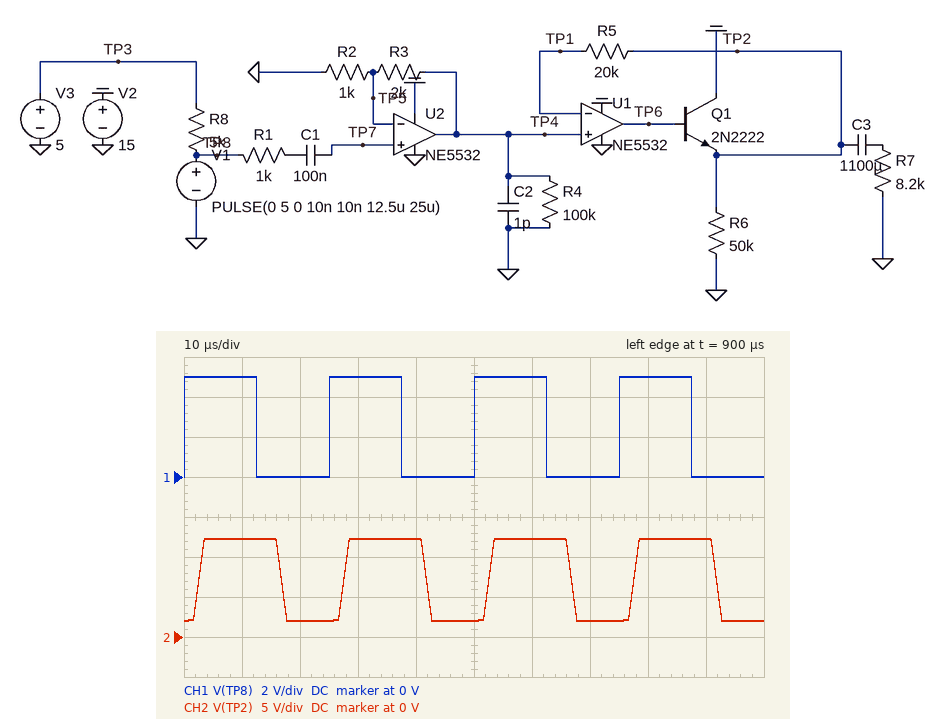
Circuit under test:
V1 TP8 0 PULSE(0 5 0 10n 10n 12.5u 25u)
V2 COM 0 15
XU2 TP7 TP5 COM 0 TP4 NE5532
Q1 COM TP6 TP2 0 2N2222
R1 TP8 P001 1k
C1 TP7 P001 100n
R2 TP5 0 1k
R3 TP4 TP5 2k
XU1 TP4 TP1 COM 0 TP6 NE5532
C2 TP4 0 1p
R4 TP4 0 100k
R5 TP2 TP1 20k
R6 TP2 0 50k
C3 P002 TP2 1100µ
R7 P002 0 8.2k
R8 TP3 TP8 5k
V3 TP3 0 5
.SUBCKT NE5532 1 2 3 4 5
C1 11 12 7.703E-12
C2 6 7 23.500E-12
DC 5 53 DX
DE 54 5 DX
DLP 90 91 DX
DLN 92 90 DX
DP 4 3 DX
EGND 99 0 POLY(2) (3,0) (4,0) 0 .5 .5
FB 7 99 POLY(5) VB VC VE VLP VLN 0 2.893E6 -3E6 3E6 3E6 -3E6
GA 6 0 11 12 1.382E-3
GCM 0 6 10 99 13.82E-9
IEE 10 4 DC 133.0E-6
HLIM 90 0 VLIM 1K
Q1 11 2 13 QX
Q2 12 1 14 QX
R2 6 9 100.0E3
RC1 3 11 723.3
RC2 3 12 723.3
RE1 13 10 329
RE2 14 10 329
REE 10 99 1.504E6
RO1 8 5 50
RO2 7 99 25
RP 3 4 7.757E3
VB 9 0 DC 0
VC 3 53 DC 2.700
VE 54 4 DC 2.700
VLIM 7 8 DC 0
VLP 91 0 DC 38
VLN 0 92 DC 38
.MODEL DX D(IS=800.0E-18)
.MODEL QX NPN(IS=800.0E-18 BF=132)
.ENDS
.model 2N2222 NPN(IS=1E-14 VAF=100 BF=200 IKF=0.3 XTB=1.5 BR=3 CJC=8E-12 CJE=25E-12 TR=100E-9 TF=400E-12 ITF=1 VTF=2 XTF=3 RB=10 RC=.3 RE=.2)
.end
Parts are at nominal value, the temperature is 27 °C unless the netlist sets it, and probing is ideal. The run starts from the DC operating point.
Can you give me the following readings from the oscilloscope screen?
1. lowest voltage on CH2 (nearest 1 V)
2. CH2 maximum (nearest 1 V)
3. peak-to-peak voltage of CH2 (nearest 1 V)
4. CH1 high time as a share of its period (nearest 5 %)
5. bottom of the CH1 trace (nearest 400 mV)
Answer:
2 V
12 V
10 V
50 %
0 V
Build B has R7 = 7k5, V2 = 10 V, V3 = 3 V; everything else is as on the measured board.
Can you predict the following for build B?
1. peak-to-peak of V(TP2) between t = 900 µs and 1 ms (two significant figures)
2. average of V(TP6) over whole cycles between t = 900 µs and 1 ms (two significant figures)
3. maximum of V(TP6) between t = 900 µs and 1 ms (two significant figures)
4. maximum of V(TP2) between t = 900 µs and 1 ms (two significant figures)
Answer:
5.3 V
5.7 V
8.0 V
7.3 V
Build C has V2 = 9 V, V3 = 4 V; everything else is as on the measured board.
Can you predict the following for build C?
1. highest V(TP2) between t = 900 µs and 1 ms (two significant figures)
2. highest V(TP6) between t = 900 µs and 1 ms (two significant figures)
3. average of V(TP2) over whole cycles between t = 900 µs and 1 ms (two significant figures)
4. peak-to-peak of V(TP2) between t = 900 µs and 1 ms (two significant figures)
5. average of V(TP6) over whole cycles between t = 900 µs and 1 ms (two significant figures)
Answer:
6.3 V
7.0 V
4.5 V
4.3 V
5.1 V
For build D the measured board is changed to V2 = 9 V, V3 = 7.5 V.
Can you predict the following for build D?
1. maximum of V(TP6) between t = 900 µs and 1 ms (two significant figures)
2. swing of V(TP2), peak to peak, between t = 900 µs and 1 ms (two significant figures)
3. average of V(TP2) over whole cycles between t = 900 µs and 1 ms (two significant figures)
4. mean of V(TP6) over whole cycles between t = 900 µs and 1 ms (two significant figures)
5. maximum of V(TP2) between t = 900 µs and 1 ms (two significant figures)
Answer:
7.0 V
4.3 V
4.5 V
5.1 V
6.3 V
